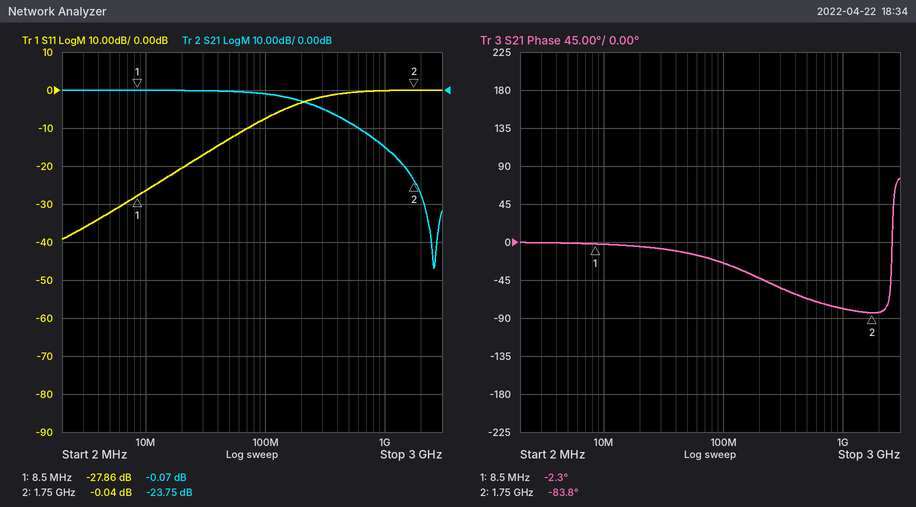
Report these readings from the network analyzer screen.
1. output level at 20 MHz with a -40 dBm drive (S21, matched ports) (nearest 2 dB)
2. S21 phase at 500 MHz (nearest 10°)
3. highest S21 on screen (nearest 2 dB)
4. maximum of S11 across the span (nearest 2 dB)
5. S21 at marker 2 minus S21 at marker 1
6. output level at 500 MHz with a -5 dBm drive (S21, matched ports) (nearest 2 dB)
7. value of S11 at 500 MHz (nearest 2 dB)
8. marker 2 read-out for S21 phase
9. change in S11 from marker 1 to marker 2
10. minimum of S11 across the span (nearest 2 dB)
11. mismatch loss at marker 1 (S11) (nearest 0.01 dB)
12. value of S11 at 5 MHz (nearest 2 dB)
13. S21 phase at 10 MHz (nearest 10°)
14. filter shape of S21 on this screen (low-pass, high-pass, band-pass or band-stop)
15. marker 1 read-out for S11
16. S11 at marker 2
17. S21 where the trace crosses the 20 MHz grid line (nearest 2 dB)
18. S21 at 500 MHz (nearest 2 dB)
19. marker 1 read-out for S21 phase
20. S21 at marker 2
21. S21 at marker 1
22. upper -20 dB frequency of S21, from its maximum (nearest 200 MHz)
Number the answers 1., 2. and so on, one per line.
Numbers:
1. -40 dBm
2. -70°
3. 0 dB
4. 0 dB
5. -23.68 dB
6. -14 dBm
7. 0 dB
8. -83.8°
9. 27.82 dB
10. -40 dB
11. 0.01 dB
12. -32 dB
13. 0°
14. low-pass
15. -27.86 dB
16. -0.04 dB
17. 0 dB
18. -8 dB
19. -2.3°
20. -23.75 dB
21. -0.07 dB
22. 1.4 GHz
